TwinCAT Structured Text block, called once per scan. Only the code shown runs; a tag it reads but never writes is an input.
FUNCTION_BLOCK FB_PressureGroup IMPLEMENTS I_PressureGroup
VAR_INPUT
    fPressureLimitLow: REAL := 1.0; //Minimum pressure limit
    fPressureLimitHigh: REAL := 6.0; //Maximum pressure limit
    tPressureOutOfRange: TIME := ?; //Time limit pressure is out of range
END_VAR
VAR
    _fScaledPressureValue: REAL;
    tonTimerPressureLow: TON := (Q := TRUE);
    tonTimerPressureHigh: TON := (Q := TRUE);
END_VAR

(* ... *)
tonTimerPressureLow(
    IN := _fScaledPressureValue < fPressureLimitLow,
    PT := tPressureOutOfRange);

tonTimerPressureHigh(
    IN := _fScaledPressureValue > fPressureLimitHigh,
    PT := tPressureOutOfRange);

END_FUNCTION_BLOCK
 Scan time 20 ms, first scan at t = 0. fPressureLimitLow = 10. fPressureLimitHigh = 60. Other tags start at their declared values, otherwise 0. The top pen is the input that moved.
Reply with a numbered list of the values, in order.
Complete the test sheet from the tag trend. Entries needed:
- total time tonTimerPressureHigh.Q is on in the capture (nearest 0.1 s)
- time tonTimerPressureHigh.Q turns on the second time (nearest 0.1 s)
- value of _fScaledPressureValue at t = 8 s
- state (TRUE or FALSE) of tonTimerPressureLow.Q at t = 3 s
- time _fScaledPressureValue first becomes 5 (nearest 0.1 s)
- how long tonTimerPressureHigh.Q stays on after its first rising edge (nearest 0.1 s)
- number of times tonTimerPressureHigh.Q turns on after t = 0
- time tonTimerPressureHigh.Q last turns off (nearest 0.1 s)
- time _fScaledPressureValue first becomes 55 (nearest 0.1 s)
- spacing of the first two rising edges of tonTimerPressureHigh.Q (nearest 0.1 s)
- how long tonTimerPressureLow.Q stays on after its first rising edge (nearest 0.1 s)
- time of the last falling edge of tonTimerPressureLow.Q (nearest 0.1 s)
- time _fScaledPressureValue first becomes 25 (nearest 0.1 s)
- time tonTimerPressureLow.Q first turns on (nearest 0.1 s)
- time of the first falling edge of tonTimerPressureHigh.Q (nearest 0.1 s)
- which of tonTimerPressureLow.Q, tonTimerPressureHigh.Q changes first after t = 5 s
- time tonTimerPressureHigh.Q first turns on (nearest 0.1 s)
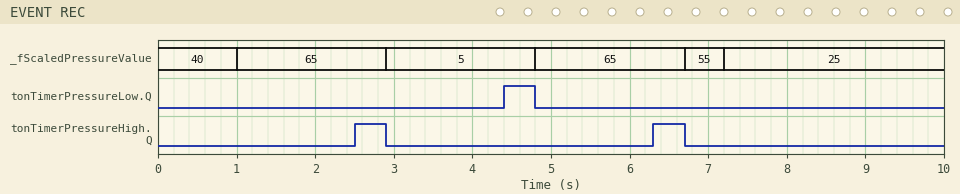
1. 0.8 s
2. 6.3 s
3. 25
4. FALSE
5. 2.9 s
6. 0.4 s
7. 2
8. 6.7 s
9. 6.7 s
10. 3.8 s
11. 0.4 s
12. 4.8 s
13. 7.2 s
14. 4.4 s
15. 2.9 s
16. tonTimerPressureHigh.Q
17. 2.5 s
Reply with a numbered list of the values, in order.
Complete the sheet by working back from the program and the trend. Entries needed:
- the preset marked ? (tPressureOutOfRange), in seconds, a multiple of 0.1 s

1. 1.5 s
